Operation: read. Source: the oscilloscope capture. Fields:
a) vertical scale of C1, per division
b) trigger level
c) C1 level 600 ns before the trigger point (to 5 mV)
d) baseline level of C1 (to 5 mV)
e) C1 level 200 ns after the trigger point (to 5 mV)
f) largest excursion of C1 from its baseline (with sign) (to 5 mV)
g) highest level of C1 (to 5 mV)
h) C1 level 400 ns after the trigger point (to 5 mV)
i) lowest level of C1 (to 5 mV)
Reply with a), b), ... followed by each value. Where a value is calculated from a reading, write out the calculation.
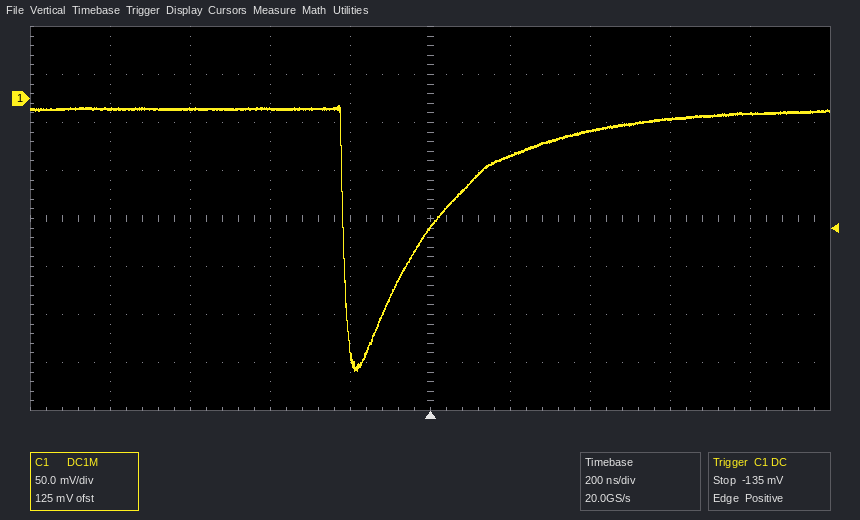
a) 50 mV
b) -135 mV
c) -10 mV
d) -10 mV
e) -60 mV
f) -285 mV − (-10 mV) = -275 mV
g) -5 mV
h) -35 mV
i) -285 mV
